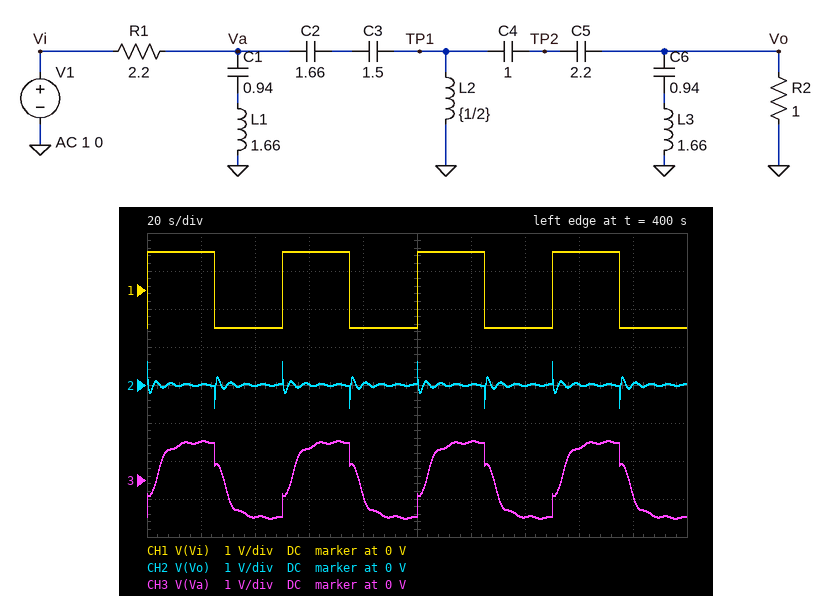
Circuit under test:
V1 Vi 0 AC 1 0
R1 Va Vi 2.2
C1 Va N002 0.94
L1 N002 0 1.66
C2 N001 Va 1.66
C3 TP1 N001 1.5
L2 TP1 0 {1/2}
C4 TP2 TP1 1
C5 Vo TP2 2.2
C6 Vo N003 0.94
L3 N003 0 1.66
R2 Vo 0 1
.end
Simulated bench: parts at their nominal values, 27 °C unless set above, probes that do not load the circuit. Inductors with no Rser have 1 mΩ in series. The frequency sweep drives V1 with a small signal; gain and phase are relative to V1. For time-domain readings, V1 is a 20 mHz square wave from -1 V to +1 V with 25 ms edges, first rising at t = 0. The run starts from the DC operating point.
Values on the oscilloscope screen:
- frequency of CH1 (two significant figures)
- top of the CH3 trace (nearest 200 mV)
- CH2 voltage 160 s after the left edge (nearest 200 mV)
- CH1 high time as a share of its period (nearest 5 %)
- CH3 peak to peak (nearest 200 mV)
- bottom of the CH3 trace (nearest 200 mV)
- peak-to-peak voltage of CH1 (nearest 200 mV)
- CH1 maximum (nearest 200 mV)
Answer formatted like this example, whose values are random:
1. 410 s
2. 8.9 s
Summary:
1. 20 mHz
2. 1.0 V
3. 0 V
4. 50 %
5. 2.0 V
6. -1.0 V
7. 2.0 V
8. 1.0 V
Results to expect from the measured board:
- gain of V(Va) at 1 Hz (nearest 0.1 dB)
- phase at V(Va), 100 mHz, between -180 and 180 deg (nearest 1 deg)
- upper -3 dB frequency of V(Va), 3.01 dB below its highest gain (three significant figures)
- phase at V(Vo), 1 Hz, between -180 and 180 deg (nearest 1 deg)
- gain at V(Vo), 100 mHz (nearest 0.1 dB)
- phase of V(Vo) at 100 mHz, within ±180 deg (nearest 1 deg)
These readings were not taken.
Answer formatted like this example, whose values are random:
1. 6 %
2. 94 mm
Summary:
1. -10.3 dB
2. -78 deg
3. 39.2 mHz
4. 28 deg
5. -41.3 dB
6. 128 deg
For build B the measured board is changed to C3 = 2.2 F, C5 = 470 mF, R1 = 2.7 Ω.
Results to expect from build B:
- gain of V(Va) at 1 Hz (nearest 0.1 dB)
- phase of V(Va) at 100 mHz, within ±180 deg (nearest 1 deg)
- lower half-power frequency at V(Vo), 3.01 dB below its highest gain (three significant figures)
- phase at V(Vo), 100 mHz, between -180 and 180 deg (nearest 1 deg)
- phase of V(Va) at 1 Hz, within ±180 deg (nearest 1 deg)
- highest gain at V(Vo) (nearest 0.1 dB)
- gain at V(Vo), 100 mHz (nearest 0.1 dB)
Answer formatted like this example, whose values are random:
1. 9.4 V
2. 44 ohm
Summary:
1. -10.3 dB
2. -81 deg
3. 291 mHz
4. 129 deg
5. -3 deg
6. -10.8 dB
7. -48.0 dB
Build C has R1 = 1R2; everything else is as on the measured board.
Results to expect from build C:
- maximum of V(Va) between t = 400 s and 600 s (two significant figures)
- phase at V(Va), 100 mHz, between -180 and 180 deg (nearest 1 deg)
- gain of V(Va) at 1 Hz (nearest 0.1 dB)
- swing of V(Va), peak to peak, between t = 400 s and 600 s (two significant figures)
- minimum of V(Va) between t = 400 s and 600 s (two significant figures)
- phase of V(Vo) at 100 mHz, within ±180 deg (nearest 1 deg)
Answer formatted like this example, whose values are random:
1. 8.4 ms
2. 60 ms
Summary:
1. 1.1 V
2. -69 deg
3. -7.0 dB
4. 2.2 V
5. -1.1 V
6. 137 deg
